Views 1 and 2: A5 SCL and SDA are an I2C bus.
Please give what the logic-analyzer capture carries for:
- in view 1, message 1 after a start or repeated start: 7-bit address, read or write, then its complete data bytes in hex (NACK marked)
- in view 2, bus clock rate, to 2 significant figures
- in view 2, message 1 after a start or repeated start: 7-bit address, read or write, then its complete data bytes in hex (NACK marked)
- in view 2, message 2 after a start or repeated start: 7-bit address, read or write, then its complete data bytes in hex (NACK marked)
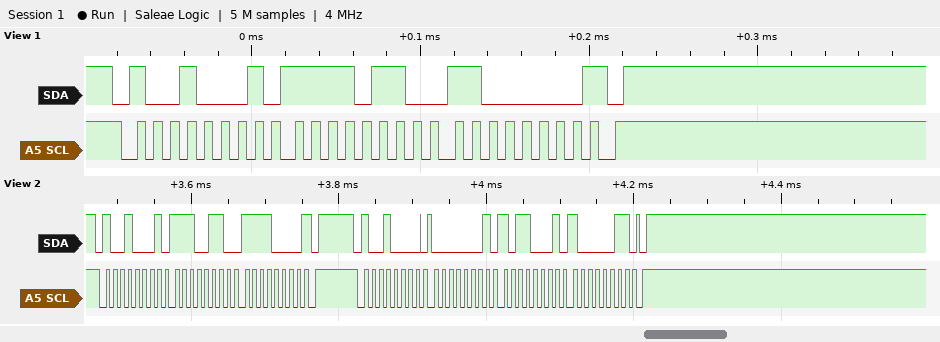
0x48 read: F6 C0 NACK
100 kHz
0x48 read: E6 F0 NACK
0x48 write: 01 B1 83
